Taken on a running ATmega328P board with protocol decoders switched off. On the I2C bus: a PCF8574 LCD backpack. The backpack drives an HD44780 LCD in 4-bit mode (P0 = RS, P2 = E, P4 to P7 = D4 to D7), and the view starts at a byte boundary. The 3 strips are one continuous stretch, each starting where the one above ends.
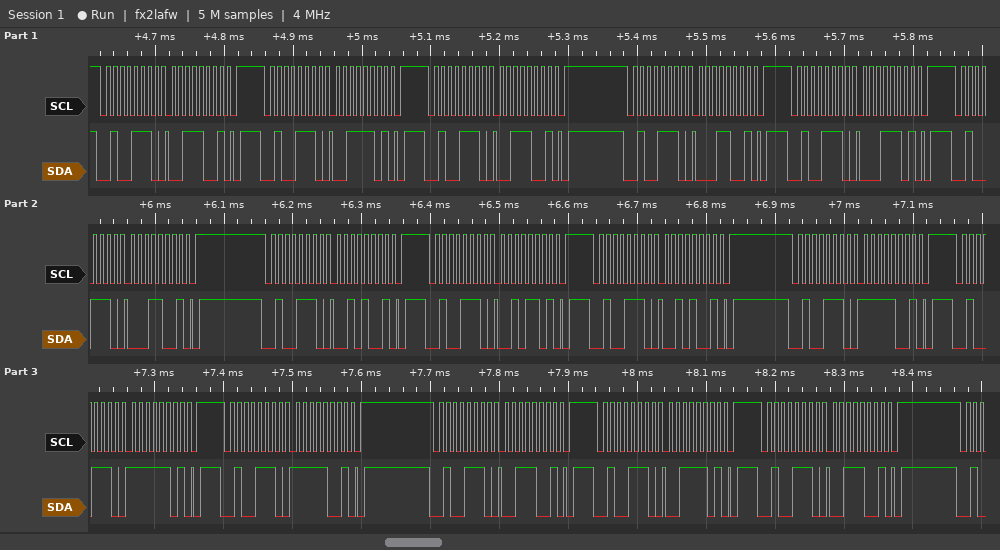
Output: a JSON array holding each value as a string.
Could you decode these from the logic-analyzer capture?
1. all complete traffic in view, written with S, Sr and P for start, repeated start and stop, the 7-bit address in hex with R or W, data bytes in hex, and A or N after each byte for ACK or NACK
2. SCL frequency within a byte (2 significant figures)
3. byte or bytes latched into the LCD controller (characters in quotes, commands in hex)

["S 27W A 39 A P S 27W A 3D A P S 27W A 39 A P S 27W A 19 A P S 27W A 1D A P S 27W A 19 A P S 27W A 29 A P S 27W A 2D A P S 27W A 29 A P S 27W A F9 A P S 27W A FD A P S 27W A F9 A P S 27W A 39 A P S 27W A 3D A P S 27W A 39 A P", "100 kHz", "'1' '/'"]
